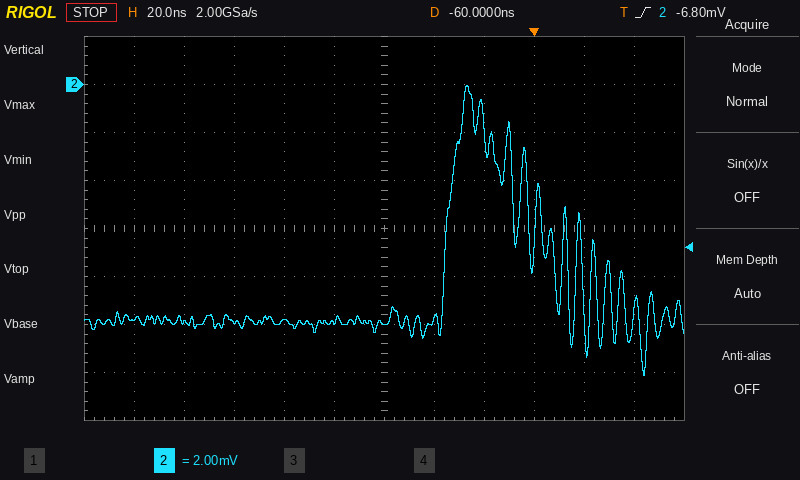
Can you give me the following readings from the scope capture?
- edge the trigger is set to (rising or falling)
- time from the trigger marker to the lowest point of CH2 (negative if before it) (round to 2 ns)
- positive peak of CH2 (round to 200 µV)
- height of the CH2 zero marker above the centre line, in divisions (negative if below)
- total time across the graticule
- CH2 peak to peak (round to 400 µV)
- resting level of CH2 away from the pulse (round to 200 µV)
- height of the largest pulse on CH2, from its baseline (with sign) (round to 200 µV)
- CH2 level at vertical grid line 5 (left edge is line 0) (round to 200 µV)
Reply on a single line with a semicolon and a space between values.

rising; +44 ns; 0.0 mV; +3.0 div; 240 ns; 12.0 mV; -9.8 mV; +9.8 mV; -9.8 mV
